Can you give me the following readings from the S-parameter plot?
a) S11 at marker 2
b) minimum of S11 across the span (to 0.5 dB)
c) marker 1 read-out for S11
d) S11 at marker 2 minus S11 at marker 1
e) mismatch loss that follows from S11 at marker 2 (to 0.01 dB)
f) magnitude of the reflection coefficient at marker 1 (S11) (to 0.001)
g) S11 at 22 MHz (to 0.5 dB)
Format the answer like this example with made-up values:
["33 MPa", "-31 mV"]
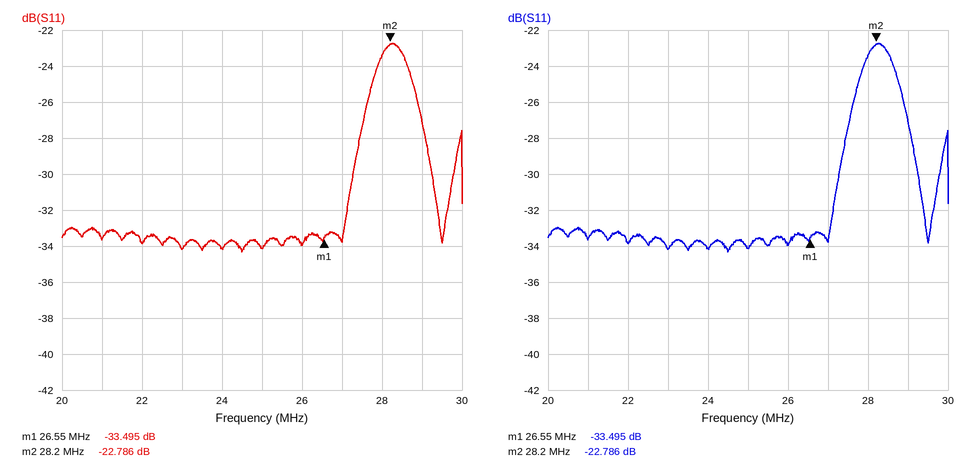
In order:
["-22.786 dB", "-34.5 dB", "-33.495 dB", "10.709 dB", "0.02 dB", "0.021", "-34.0 dB"]
